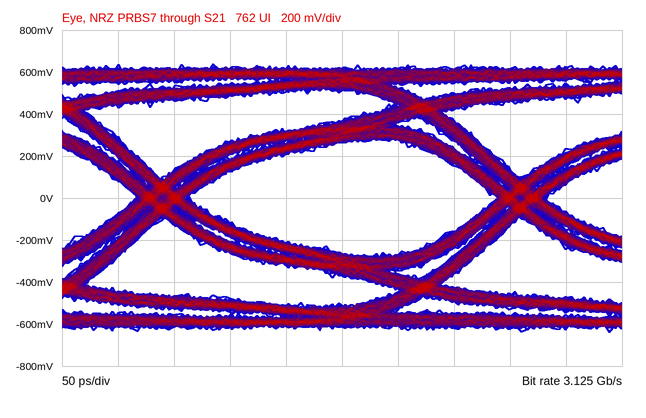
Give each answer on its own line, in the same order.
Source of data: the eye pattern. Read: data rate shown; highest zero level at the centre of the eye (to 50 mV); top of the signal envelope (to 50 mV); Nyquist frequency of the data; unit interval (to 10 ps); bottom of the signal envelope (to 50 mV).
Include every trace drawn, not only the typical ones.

3.125 Gb/s
-250 mV
650 mV
1.5625 GHz
320 ps
-650 mV
